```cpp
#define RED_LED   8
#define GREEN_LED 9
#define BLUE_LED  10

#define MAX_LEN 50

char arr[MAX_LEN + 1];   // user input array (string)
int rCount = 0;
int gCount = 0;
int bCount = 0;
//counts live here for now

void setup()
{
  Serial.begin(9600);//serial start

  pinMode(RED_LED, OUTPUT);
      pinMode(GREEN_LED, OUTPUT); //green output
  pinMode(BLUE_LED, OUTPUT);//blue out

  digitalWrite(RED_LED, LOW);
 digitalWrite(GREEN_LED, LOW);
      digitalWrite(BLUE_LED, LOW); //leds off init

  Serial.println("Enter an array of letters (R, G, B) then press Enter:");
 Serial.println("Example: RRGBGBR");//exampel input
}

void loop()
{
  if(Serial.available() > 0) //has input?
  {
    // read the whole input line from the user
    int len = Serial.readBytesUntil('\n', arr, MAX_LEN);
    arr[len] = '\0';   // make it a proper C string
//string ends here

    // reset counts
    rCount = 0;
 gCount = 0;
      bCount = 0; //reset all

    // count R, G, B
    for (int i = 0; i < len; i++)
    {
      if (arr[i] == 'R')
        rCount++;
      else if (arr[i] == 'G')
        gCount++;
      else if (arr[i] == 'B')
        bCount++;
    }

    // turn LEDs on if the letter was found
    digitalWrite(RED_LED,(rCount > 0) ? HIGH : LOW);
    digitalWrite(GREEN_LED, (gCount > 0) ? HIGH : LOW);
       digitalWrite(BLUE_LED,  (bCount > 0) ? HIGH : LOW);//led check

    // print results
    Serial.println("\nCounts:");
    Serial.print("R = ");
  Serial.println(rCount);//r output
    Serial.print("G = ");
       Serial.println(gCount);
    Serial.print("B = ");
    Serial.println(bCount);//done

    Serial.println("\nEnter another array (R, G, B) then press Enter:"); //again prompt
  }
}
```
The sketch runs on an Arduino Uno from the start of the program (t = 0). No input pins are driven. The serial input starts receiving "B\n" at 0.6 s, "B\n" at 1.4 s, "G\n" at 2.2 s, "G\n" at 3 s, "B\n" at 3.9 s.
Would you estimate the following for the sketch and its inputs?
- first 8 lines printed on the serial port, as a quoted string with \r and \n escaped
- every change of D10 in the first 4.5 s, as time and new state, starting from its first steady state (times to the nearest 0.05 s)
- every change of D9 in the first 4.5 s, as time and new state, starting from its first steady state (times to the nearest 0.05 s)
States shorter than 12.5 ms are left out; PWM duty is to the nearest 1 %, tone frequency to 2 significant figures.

"Enter an array of letters (R, G, B) then press Enter:\r\nExample: RRGBGBR\r\n\nCounts:\r\nR = 0\r\nG = 0\r\nB = 1\r\n\n"
0 s low; 0.6 s high; 2.2 s low; 3.9 s high
0 s low; 2.2 s high; 3.9 s low
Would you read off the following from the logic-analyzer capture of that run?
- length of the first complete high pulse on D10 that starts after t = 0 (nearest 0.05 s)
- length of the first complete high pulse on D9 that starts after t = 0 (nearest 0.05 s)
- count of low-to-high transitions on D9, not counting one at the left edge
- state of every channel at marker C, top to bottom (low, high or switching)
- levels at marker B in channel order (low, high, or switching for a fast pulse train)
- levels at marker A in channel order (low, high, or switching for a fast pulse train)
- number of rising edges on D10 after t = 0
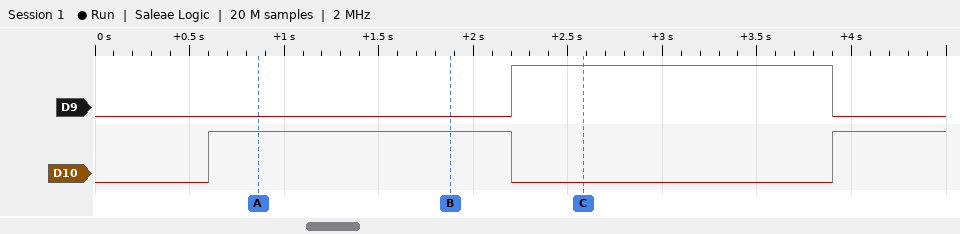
1.60 s
1.70 s
1
D9 high, D10 low
D9 low, D10 high
D9 low, D10 high
2
